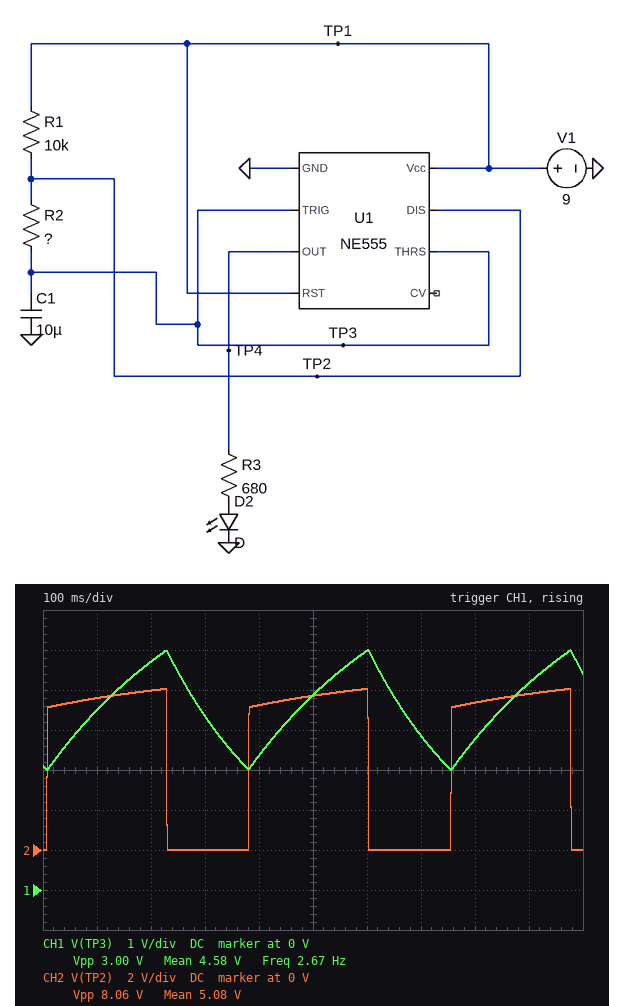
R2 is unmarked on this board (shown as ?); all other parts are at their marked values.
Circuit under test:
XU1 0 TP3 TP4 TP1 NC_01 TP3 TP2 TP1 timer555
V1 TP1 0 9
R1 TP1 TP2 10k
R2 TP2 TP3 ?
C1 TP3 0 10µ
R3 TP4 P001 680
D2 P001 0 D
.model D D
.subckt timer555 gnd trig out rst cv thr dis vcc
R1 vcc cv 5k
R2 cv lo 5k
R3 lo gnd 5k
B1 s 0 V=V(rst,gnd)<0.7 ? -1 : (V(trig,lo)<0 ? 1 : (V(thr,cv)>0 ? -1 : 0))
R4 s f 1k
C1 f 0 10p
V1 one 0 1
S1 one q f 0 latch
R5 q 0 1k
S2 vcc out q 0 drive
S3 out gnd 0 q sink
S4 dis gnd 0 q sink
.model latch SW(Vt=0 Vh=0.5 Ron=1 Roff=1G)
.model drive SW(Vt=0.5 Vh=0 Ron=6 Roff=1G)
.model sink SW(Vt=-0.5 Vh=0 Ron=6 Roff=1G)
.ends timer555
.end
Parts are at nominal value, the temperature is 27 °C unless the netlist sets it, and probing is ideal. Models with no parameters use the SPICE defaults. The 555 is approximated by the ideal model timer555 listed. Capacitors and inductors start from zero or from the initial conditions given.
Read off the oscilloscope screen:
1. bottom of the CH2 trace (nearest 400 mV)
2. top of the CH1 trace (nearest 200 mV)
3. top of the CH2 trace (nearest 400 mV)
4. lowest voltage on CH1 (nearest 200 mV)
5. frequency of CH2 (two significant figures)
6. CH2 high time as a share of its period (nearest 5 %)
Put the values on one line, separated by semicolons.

0 V; 6.0 V; 8.0 V; 3.0 V; 2.7 Hz; 60 %
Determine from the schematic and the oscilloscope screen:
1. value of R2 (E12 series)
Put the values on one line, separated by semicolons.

22 kΩ
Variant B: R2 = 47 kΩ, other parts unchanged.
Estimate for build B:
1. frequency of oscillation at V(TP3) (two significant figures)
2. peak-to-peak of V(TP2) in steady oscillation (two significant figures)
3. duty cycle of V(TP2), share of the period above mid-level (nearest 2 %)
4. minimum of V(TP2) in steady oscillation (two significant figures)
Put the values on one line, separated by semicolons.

1.4 Hz; 8.5 V; 54 %; 5.8 mV
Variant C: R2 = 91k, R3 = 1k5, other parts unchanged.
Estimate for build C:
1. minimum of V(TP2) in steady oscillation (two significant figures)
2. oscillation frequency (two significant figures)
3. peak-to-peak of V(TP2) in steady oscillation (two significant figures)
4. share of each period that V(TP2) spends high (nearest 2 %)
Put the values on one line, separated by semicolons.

5.6 mV; 750 mHz; 8.7 V; 52 %
